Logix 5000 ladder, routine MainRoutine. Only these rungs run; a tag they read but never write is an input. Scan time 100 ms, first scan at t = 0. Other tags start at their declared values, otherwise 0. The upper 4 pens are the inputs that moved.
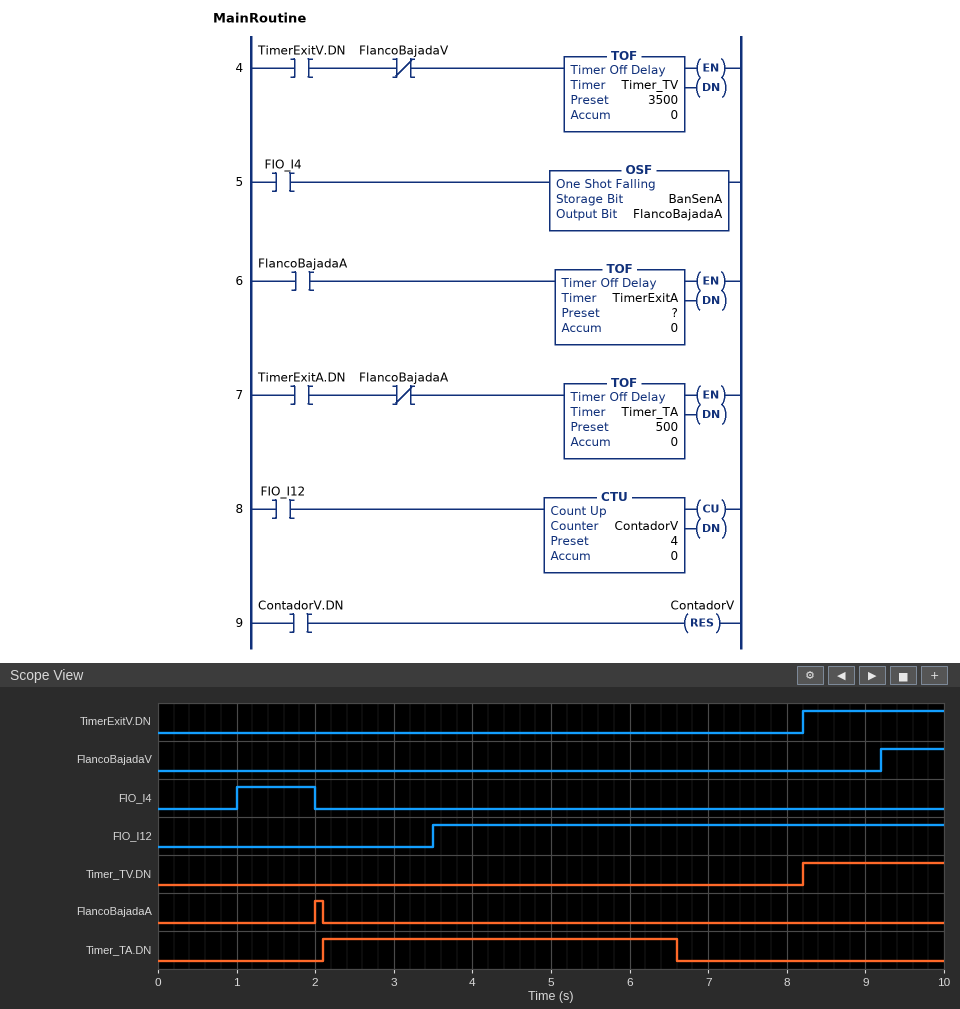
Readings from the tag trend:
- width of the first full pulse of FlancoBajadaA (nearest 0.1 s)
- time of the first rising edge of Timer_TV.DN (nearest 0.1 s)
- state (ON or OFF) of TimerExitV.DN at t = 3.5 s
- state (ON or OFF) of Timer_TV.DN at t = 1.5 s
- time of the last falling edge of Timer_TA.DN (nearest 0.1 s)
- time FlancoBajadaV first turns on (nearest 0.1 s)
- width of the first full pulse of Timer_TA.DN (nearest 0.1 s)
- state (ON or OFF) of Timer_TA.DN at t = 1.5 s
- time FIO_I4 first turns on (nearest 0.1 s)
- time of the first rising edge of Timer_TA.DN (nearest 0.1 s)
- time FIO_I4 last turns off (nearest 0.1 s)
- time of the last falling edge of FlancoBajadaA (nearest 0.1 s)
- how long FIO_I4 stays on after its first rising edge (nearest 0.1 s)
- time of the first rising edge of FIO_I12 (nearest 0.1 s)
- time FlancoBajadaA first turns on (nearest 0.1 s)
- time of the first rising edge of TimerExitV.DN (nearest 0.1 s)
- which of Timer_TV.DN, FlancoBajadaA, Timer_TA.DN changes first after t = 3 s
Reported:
0.1 s
8.2 s
OFF
OFF
6.6 s
9.2 s
4.5 s
OFF
1.0 s
2.1 s
2.0 s
2.1 s
1.0 s
3.5 s
2.0 s
8.2 s
Timer_TA.DN
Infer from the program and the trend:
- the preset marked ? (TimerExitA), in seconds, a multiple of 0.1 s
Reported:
4.0 s
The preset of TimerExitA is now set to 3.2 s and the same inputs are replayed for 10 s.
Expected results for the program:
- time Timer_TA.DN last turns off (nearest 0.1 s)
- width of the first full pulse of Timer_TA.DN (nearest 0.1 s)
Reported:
5.8 s
3.7 s
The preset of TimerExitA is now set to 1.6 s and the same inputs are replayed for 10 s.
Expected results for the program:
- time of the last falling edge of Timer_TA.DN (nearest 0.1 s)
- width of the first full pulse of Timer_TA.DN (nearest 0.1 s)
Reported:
4.2 s
2.1 s
